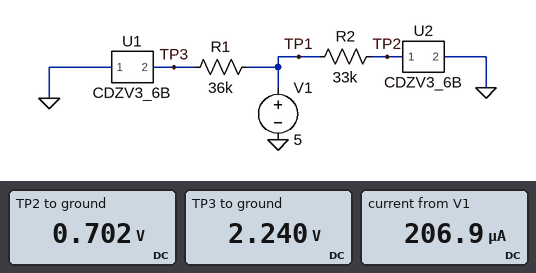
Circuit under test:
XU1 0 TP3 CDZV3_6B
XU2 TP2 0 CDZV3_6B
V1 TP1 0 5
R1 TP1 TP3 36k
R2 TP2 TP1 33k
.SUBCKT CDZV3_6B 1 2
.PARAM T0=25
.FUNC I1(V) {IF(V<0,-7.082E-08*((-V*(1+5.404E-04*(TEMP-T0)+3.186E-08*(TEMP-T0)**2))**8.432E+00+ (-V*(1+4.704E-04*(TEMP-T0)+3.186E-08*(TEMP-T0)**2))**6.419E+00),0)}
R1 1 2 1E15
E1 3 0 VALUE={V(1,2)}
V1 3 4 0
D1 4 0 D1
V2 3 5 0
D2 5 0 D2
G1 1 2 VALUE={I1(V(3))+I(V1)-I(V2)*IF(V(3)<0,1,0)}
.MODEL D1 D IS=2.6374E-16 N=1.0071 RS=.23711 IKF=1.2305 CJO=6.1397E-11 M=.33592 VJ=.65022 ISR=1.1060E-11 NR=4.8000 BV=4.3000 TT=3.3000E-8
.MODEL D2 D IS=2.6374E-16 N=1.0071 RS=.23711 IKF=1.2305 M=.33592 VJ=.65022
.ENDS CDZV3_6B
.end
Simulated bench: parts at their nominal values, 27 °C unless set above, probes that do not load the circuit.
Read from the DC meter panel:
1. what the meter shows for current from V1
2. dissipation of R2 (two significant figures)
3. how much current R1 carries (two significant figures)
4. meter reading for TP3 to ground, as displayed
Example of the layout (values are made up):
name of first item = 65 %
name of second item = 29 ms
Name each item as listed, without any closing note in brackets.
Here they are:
what the meter shows for current from V1 = 206.9 µA
dissipation of R2 = 560 µW
how much current R1 carries = 77 µA
meter reading for TP3 to ground, as displayed = 2.240 V
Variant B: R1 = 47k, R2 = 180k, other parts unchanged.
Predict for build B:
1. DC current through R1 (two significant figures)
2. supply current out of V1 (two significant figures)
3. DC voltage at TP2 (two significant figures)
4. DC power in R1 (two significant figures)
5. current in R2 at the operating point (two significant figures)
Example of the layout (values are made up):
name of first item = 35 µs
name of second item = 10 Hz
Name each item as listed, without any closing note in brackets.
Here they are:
DC current through R1 = 60 µA
supply current out of V1 = 84 µA
DC voltage at TP2 = 660 mV
DC power in R1 = 170 µW
current in R2 at the operating point = 24 µA
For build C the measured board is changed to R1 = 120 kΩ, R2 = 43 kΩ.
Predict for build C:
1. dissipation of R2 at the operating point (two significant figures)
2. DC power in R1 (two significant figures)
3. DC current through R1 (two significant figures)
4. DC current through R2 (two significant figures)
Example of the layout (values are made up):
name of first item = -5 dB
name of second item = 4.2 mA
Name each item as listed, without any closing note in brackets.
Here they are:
dissipation of R2 at the operating point = 430 µW
DC power in R1 = 77 µW
DC current through R1 = 25 µA
DC current through R2 = 100 µA
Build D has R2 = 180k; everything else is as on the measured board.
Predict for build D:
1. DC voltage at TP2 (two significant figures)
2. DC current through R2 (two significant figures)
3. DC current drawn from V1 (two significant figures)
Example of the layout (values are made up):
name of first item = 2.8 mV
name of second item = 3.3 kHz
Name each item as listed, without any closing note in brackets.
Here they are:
DC voltage at TP2 = 660 mV
DC current through R2 = 24 µA
DC current drawn from V1 = 100 µA
